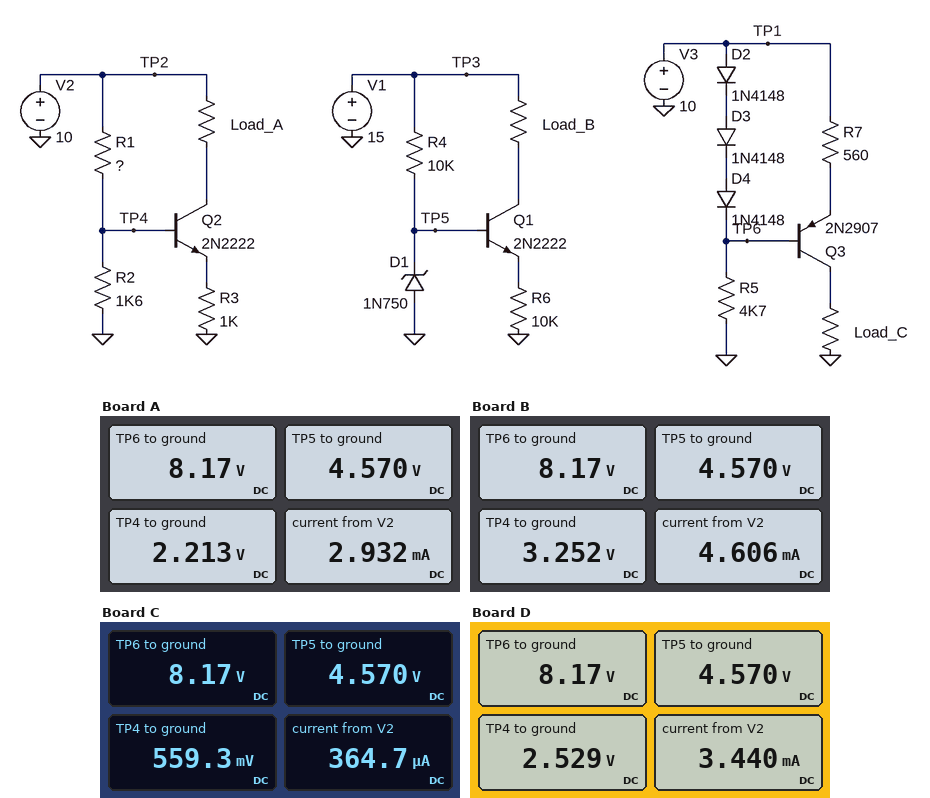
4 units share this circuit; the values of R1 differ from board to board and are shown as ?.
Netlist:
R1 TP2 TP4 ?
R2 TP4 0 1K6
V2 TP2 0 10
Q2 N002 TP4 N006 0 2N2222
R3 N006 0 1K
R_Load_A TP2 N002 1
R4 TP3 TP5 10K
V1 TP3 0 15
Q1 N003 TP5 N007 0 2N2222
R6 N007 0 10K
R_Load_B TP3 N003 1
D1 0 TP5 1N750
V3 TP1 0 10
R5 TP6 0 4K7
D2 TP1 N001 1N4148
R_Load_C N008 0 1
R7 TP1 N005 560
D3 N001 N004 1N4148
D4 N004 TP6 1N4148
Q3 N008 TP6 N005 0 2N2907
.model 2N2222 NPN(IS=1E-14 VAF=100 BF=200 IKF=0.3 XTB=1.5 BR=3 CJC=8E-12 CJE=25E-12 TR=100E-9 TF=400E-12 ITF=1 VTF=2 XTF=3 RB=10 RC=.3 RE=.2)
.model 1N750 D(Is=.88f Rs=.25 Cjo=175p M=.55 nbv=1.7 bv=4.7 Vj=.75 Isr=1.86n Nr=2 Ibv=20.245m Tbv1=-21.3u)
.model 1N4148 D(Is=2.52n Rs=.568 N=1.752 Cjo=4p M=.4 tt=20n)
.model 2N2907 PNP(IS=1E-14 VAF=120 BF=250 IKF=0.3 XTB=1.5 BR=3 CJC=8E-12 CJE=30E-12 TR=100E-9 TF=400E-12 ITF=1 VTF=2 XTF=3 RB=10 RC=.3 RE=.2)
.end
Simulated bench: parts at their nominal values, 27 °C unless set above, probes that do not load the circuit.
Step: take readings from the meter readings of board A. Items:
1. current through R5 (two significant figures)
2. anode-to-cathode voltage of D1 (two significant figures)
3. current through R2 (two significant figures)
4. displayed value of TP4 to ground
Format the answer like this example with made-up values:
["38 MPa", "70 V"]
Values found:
["1.7 mA", "-4.6 V", "1.4 mA", "2.213 V"]
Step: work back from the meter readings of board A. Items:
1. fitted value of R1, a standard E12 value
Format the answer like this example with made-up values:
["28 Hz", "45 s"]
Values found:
["5.6 kΩ"]
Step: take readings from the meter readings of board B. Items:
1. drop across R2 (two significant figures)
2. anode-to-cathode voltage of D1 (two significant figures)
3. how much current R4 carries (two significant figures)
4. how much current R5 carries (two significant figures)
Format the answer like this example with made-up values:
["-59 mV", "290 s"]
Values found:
["3.3 V", "-4.6 V", "1.0 mA", "1.7 mA"]
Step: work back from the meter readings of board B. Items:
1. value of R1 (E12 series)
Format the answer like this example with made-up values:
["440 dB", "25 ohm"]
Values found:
["3.3 kΩ"]
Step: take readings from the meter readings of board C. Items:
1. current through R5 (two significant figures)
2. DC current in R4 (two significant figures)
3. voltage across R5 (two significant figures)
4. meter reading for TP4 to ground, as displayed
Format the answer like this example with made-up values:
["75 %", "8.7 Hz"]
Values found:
["1.7 mA", "1.0 mA", "8.2 V", "559.3 mV"]
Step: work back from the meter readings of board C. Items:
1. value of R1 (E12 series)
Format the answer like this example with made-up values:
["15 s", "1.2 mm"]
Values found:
["27 kΩ"]
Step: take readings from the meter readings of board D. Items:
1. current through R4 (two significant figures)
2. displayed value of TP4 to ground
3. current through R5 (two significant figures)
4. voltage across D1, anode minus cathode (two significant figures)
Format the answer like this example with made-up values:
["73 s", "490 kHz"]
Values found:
["1.0 mA", "2.529 V", "1.7 mA", "-4.6 V"]
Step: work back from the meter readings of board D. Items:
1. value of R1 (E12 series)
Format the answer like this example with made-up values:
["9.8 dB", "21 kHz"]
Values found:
["4.7 kΩ"]
